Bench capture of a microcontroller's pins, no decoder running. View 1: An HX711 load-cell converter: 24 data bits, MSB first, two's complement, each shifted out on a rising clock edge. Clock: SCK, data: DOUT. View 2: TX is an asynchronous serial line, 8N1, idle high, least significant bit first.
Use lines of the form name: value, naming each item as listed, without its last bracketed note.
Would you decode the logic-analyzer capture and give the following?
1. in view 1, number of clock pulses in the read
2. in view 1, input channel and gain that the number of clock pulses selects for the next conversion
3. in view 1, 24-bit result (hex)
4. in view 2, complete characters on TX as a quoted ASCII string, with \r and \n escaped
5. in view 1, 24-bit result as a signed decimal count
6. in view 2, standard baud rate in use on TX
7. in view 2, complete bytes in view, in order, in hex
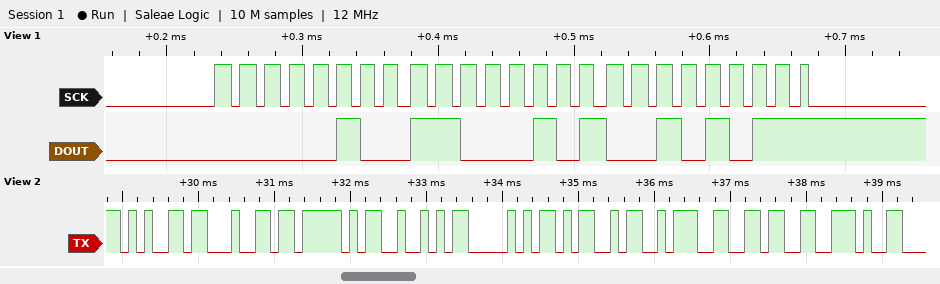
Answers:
in view 1, number of clock pulses in the read: 25
in view 1, input channel and gain that the number of clock pulses selects for the next conversion: channel A, gain 128
in view 1, 24-bit result: 0x04C52B
in view 2, complete characters on TX as a quoted ASCII string, with \r and \n escaped: "ed_RPM:6."
in view 1, 24-bit result as a signed decimal count: 312619
in view 2, standard baud rate in use on TX: 9600 baud
in view 2, complete bytes in view, in order, in hex: 65 64 5F 52 50 4D 3A 36 2E
